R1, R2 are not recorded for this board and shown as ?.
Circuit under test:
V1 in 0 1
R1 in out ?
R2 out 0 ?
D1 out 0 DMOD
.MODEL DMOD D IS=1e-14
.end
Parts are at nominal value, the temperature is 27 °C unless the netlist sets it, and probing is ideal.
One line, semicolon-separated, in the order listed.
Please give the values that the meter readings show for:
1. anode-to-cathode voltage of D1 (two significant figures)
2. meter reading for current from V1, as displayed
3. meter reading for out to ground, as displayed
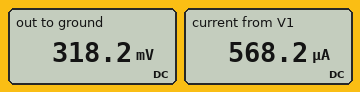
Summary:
320 mV; 568.2 µA; 318.2 mV
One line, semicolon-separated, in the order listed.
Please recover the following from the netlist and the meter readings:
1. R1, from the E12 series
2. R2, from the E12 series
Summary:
1.2 kΩ; 560 Ω
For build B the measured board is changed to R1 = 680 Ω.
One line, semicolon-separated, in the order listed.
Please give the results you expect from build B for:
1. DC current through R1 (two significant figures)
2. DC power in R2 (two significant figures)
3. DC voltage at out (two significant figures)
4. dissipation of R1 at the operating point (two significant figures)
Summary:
810 µA; 360 µW; 450 mV; 440 µW
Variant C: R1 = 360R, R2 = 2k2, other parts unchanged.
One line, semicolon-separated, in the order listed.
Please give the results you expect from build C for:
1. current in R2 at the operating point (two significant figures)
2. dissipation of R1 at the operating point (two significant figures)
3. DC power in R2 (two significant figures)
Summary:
290 µA; 350 µW; 190 µW
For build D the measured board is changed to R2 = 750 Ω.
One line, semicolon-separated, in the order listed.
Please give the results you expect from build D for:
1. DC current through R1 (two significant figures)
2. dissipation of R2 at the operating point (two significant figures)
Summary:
510 µA; 200 µW
